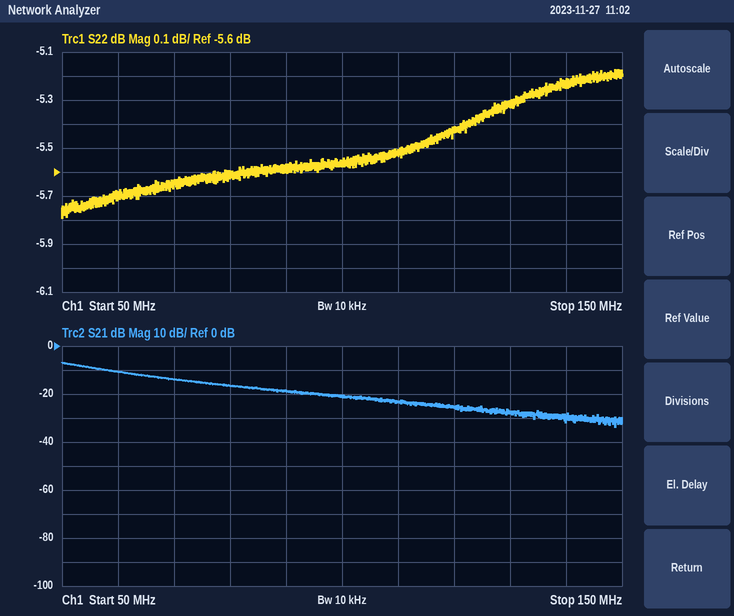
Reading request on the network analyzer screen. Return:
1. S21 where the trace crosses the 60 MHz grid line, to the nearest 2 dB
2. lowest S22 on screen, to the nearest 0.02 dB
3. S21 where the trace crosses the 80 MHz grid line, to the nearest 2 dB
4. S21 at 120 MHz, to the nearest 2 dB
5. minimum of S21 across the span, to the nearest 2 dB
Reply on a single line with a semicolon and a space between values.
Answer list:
-10 dB; -5.80 dB; -16 dB; -26 dB; -34 dB
